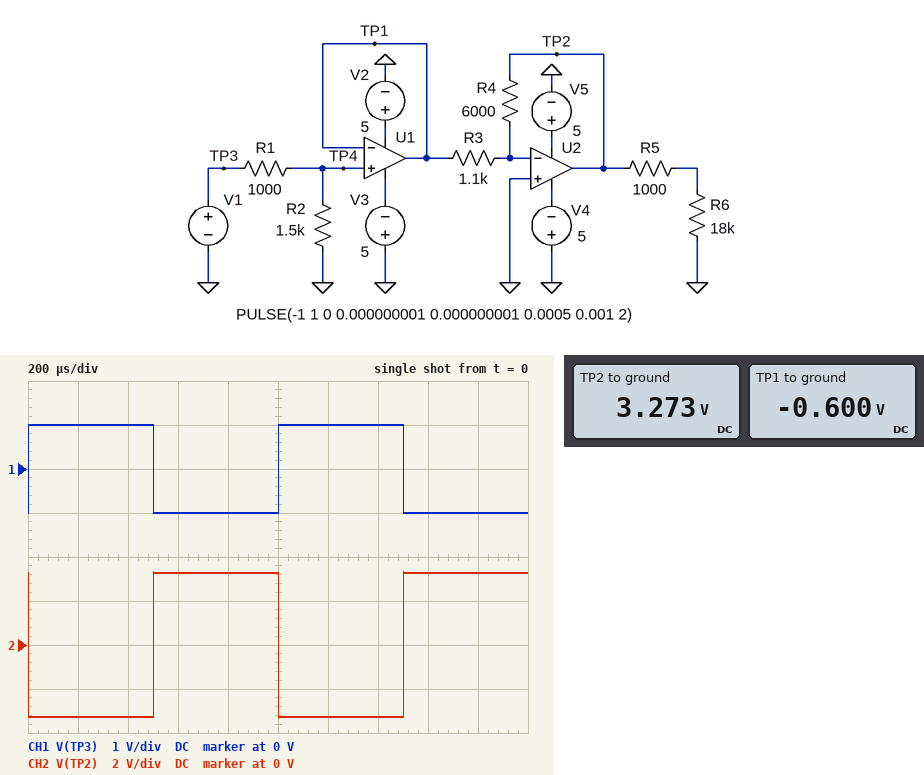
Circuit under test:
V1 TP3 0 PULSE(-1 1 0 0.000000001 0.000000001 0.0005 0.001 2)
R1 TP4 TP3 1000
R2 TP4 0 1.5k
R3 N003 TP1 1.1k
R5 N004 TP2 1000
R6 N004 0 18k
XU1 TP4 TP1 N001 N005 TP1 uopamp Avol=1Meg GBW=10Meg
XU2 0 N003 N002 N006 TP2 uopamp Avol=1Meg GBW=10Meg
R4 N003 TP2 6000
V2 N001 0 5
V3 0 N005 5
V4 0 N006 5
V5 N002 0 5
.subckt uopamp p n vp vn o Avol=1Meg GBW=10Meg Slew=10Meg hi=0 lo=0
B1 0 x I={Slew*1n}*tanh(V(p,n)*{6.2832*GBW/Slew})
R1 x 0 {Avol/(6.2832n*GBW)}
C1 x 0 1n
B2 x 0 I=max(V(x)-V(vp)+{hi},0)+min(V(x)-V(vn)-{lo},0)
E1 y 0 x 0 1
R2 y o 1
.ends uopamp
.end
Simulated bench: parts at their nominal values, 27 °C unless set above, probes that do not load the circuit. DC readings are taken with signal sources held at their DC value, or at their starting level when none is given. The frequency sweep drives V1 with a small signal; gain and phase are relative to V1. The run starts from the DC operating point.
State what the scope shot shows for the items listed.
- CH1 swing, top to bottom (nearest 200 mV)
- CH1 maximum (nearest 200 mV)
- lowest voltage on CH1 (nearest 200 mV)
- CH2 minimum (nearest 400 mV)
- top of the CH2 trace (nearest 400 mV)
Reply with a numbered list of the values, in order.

1. 2.0 V
2. 1.0 V
3. -1.0 V
4. -3.2 V
5. 3.2 V
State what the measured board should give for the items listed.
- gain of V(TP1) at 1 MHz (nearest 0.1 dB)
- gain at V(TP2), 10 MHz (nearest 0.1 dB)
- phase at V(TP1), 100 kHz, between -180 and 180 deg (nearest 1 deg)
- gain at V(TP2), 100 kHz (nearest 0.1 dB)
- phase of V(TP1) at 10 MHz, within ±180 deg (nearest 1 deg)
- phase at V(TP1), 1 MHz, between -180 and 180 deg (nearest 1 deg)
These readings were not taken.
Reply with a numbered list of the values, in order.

1. -4.5 dB
2. -9.0 dB
3. -1 deg
4. 10.3 dB
5. -45 deg
6. -6 deg
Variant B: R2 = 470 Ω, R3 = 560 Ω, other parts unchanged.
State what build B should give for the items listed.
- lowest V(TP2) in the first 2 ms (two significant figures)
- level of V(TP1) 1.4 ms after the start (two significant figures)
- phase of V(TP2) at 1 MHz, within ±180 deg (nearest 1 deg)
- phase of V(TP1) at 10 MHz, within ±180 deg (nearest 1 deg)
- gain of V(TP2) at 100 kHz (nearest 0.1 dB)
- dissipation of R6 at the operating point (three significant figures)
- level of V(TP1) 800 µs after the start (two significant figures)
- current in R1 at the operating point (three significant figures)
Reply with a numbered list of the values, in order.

1. -3.4 V
2. 320 mV
3. 125 deg
4. -45 deg
5. 10.6 dB
6. 585 µW
7. -320 mV
8. 680 µA
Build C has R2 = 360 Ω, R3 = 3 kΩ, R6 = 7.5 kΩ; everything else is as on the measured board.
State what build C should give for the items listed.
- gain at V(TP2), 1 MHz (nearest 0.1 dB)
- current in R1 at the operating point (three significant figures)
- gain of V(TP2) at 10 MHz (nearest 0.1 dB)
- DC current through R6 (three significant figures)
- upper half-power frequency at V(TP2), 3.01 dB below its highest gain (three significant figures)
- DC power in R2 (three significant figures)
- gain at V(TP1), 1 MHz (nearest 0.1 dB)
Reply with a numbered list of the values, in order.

1. -5.9 dB
2. 735 µA
3. -18.5 dB
4. 62.3 µA
5. 3.04 MHz
6. 195 µW
7. -11.6 dB
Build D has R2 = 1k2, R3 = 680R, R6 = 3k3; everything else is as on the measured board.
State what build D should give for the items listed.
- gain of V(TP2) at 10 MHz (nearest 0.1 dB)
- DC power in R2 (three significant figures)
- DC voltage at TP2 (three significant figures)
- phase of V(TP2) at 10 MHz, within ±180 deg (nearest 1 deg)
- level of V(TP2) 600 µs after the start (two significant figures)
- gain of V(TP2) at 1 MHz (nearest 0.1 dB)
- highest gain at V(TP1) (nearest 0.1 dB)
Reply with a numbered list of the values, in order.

1. -9.3 dB
2. 248 µW
3. 4.81 V
4. 51 deg
5. 4.8 V
6. 10.7 dB
7. -5.3 dB
